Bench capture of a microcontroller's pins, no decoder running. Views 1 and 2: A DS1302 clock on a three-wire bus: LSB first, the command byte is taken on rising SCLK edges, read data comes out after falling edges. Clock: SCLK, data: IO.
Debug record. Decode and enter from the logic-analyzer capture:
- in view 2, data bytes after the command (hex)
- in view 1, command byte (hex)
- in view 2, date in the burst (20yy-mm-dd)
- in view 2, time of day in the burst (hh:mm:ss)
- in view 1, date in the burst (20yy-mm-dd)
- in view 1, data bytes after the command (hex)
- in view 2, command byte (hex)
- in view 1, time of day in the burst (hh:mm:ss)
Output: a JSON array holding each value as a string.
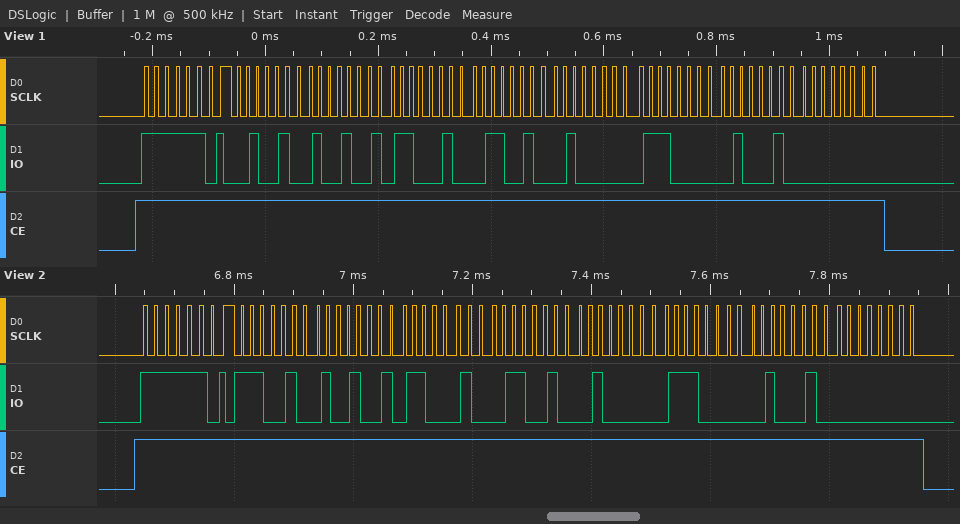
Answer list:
["27 49 23 26 02 07 22 00", "0xBF", "2022-02-26", "23:49:27", "2022-02-26", "24 49 23 26 02 07 22 00", "0xBF", "23:49:24"]
